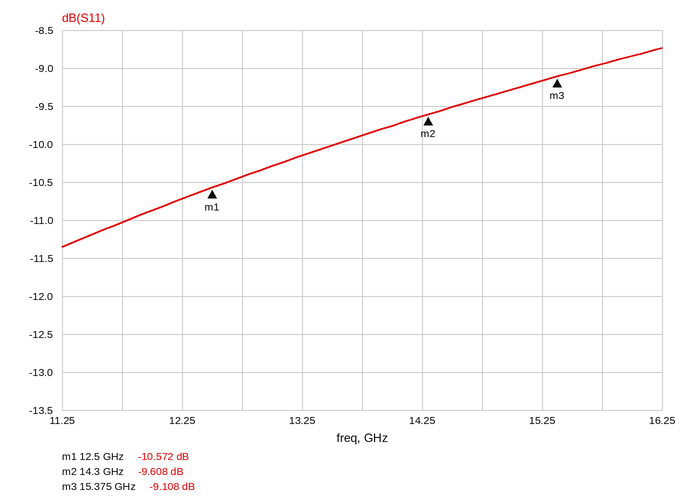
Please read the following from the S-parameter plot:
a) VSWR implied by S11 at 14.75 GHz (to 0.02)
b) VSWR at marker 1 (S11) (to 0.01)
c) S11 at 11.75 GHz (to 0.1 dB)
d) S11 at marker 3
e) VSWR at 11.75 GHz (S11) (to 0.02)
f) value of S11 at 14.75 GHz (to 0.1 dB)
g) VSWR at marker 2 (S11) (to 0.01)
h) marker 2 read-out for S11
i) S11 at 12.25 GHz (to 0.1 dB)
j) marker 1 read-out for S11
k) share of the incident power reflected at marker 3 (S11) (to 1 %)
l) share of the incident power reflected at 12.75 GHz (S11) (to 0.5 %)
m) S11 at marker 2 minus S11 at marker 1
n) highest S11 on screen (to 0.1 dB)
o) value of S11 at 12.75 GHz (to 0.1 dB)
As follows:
2.02
1.84
-11.0 dB
-9.108 dB
1.78
-9.4 dB
1.99
-9.608 dB
-10.7 dB
-10.572 dB
12 %
9.0 %
0.964 dB
-8.7 dB
-10.4 dB
